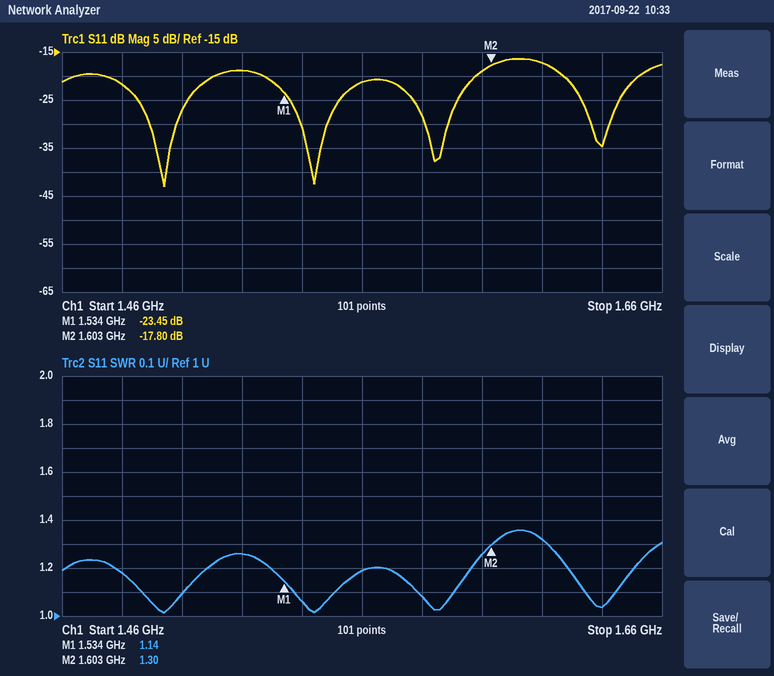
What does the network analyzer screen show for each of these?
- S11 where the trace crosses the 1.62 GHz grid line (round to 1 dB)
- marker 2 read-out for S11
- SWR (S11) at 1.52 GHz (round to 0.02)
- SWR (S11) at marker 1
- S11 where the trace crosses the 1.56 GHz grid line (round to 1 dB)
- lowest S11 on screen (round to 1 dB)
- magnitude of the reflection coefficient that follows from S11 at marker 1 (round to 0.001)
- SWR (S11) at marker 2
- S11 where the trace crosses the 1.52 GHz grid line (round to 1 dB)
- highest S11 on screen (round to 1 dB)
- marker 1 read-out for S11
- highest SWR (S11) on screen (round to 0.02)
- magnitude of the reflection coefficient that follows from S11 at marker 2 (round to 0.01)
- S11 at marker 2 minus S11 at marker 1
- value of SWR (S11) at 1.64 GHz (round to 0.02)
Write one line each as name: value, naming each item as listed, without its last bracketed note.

S11 where the trace crosses the 1.62 GHz grid line: -17 dB
marker 2 read-out for S11: -17.80 dB
SWR (S11) at 1.52 GHz: 1.26
SWR (S11) at marker 1: 1.14
S11 where the trace crosses the 1.56 GHz grid line: -21 dB
lowest S11 on screen: -43 dB
magnitude of the reflection coefficient that follows from S11 at marker 1: 0.067
SWR (S11) at marker 2: 1.30
S11 where the trace crosses the 1.52 GHz grid line: -19 dB
highest S11 on screen: -16 dB
marker 1 read-out for S11: -23.45 dB
highest SWR (S11) on screen: 1.36
magnitude of the reflection coefficient that follows from S11 at marker 2: 0.13
S11 at marker 2 minus S11 at marker 1: 5.65 dB
value of SWR (S11) at 1.64 GHz: 1.04
